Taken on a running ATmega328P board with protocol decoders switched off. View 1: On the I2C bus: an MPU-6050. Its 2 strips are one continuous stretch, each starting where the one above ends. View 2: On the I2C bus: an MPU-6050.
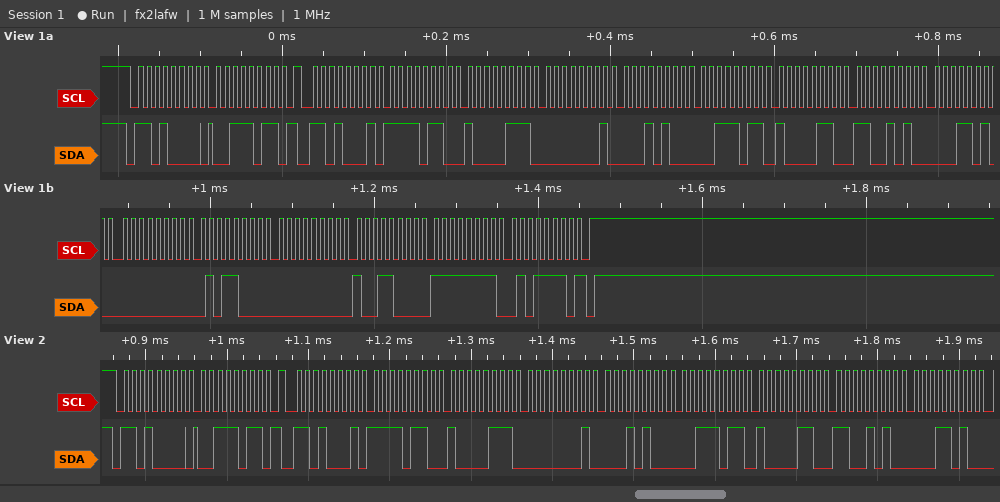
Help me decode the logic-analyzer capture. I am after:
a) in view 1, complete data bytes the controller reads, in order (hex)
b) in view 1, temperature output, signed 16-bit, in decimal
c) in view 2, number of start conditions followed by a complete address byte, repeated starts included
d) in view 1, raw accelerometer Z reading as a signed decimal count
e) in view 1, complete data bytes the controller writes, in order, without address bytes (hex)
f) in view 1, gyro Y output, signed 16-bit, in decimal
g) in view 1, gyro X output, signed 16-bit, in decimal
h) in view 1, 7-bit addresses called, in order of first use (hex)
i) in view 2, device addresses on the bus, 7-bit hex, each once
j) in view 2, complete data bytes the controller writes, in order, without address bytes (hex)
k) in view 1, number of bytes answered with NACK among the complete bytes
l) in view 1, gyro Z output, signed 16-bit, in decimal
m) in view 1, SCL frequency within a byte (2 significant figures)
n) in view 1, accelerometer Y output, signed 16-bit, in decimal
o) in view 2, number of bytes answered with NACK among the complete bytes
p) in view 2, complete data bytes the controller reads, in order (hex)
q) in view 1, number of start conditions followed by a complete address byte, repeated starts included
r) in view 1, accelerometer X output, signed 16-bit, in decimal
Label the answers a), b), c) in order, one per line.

a) F6 87 01 14 3B 86 CA 1A 00 58 00 98 FF 5E
b) -13798
c) 2
d) 15238
e) 3B
f) 152
g) 88
h) 0x68
i) 0x68
j) 3B
k) 1
l) -162
m) 100 kHz
n) 276
o) 0
p) F6 87 01 14 3B 86 CA 1A
q) 2
r) -2425
